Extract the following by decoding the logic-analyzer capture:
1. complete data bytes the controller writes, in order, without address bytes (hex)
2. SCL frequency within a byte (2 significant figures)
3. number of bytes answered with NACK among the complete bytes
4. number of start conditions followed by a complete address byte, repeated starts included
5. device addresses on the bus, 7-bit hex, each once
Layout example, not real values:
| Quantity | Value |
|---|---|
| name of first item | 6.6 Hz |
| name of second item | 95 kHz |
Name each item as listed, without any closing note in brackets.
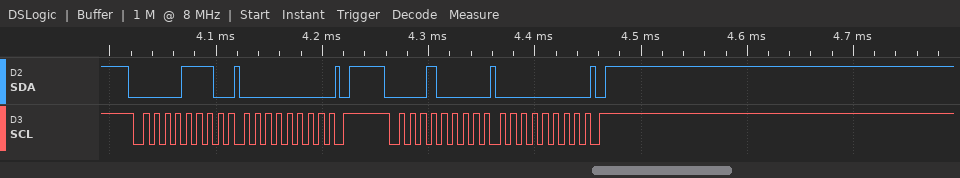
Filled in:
| Quantity | Value |
|---|---|
| complete data bytes the controller writes, in order, without address bytes | 00 00 |
| SCL frequency within a byte | 100 kHz |
| number of bytes answered with NACK among the complete bytes | 0 |
| number of start conditions followed by a complete address byte, repeated starts included | 2 |
| device addresses on the bus, 7-bit hex, each once | 0x07 0x08 |
